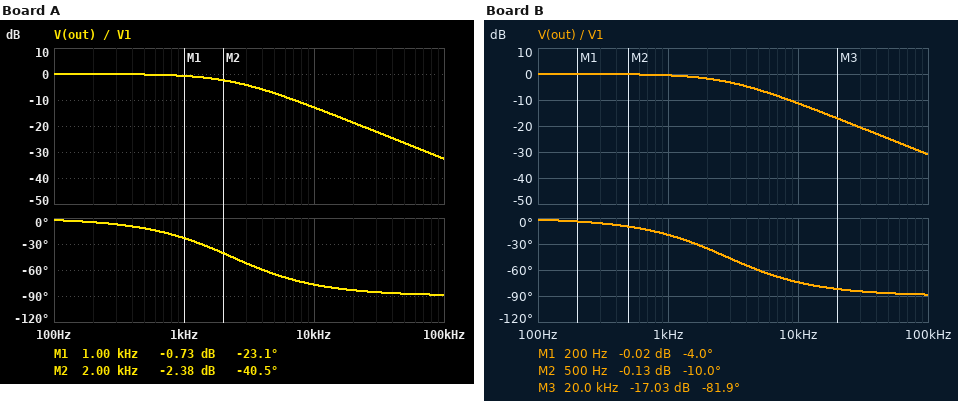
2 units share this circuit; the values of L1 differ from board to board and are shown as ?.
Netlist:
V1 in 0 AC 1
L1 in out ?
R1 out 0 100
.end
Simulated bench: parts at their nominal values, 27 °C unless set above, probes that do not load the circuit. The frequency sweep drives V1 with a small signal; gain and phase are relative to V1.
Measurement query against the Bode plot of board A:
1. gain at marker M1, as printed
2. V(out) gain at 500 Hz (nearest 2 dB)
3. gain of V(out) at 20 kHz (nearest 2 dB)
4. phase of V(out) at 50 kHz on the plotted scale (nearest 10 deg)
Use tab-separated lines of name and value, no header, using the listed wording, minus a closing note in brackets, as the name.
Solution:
gain at marker M1, as printed	-0.73 dB
V(out) gain at 500 Hz	0 dB
gain of V(out) at 20 kHz	-18 dB
phase of V(out) at 50 kHz on the plotted scale	-90 deg
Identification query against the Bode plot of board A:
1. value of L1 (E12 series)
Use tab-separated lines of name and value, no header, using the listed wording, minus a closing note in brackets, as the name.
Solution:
value of L1	6.8 mH
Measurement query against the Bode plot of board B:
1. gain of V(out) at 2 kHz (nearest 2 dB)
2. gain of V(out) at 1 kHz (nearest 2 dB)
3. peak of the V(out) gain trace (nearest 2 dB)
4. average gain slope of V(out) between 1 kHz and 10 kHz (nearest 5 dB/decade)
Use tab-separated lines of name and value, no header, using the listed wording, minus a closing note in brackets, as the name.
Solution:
gain of V(out) at 2 kHz	-2 dB
gain of V(out) at 1 kHz	0 dB
peak of the V(out) gain trace	0 dB
average gain slope of V(out) between 1 kHz and 10 kHz	-10 dB/decade
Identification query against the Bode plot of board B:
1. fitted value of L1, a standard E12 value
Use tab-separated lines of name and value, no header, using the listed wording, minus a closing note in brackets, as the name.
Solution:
fitted value of L1, a standard E12 value	5.6 mH
